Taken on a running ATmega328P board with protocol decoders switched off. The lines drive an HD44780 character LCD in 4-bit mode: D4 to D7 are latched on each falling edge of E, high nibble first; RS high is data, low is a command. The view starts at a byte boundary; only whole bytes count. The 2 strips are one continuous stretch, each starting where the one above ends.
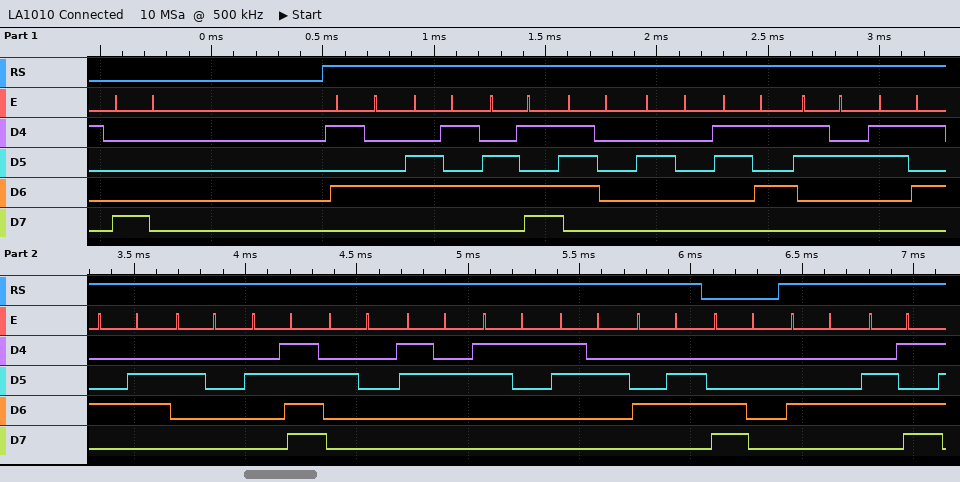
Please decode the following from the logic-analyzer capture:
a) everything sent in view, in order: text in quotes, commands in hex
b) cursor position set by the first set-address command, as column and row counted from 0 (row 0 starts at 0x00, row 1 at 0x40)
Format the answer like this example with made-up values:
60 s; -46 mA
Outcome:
0x80 "Temp 525F / 212F" 0xC0 "Dm"; column 0, row 0
